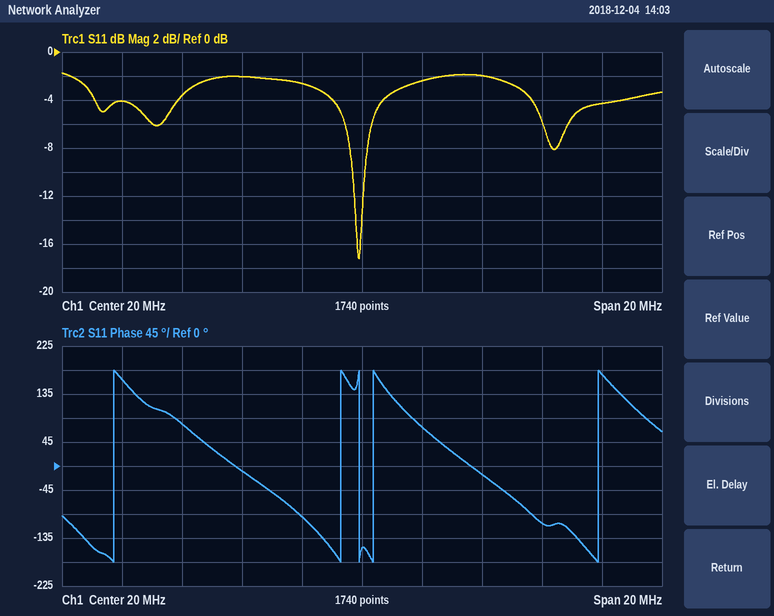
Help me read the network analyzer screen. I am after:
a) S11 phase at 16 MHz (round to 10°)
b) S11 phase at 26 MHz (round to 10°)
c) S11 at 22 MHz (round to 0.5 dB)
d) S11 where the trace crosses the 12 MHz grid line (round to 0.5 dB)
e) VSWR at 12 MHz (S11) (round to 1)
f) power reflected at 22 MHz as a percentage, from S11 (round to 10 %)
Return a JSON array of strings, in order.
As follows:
["-10°", "-110°", "-2.5 dB", "-4.0 dB", "4", "60 %"]
